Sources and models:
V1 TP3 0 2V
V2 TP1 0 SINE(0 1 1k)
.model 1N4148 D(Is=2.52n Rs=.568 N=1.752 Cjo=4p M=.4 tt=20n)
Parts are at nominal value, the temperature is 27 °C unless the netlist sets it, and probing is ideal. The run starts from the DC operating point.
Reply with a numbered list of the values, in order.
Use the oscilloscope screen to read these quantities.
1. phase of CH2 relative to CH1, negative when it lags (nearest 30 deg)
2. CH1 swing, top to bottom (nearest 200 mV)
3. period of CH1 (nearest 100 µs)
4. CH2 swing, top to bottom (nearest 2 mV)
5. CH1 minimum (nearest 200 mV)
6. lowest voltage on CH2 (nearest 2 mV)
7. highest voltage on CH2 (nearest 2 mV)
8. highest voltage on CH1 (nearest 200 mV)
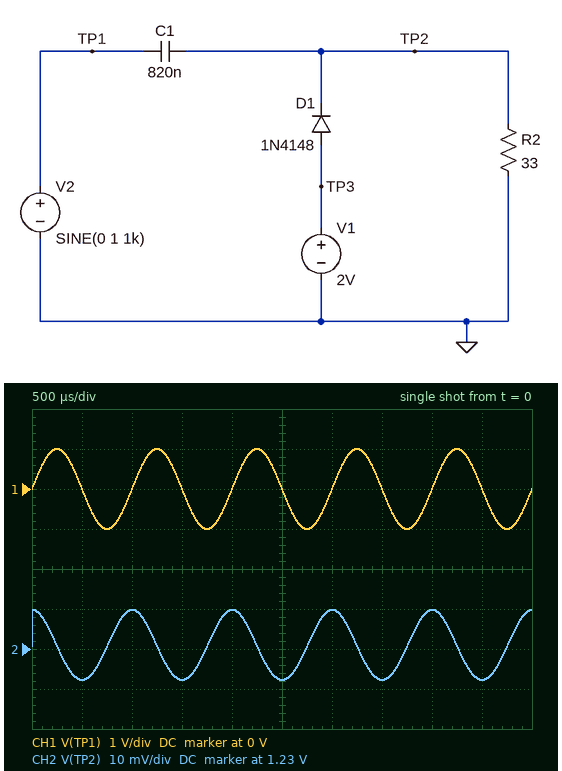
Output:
1. 90 deg
2. 2.0 V
3. 1.0 ms
4. 18 mV
5. -1.0 V
6. 1.222 V
7. 1.240 V
8. 1.0 V
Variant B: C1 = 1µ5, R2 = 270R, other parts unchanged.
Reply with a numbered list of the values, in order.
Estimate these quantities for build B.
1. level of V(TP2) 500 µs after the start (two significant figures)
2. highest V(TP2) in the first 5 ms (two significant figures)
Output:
1. 1.3 V
2. 1.8 V
